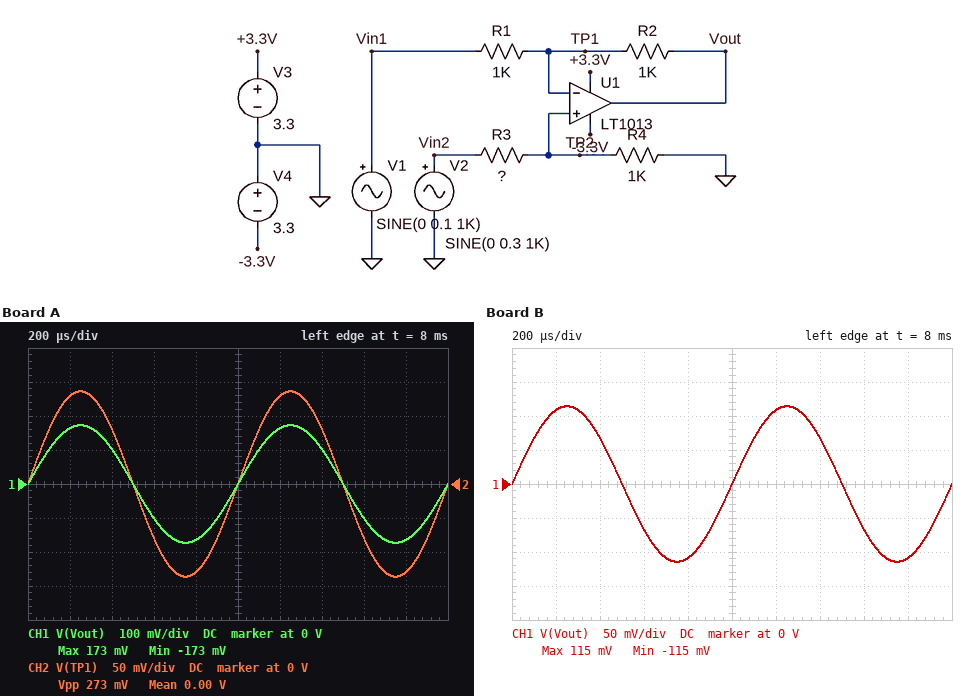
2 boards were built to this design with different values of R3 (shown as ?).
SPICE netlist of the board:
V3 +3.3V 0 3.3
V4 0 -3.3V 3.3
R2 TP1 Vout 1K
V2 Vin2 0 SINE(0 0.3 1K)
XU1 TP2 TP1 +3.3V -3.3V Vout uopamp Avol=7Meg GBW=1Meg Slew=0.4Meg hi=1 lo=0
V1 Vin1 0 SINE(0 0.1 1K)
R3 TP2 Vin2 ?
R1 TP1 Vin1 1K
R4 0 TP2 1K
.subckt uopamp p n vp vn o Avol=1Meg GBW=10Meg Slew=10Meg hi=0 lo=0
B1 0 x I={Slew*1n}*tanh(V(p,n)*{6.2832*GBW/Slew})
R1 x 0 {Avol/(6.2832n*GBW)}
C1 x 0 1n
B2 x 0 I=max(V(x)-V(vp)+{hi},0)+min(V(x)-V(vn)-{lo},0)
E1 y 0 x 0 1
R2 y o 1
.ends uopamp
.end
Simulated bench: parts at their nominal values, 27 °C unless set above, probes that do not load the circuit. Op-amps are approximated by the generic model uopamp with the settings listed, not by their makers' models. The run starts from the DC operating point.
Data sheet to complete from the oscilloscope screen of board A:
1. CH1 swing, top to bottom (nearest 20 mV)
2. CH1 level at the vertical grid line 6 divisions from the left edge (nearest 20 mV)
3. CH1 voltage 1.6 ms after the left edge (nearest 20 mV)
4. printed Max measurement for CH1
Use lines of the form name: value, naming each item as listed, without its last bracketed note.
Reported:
CH1 swing, top to bottom: 340 mV
CH1 level at the vertical grid line 6 divisions from the left edge: 160 mV
CH1 voltage 1.6 ms after the left edge: -100 mV
printed Max measurement for CH1: 173 mV
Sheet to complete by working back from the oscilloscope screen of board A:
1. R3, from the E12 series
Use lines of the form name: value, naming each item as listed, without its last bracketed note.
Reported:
R3, from the E12 series: 1.2 kΩ
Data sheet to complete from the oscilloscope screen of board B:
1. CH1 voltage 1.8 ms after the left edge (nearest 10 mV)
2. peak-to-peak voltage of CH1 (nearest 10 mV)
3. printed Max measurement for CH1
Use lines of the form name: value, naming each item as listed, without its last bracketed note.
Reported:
CH1 voltage 1.8 ms after the left edge: -110 mV
peak-to-peak voltage of CH1: 230 mV
printed Max measurement for CH1: 115 mV
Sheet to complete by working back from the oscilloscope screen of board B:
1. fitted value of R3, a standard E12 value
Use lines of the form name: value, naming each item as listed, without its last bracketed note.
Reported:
fitted value of R3, a standard E12 value: 1.8 kΩ
